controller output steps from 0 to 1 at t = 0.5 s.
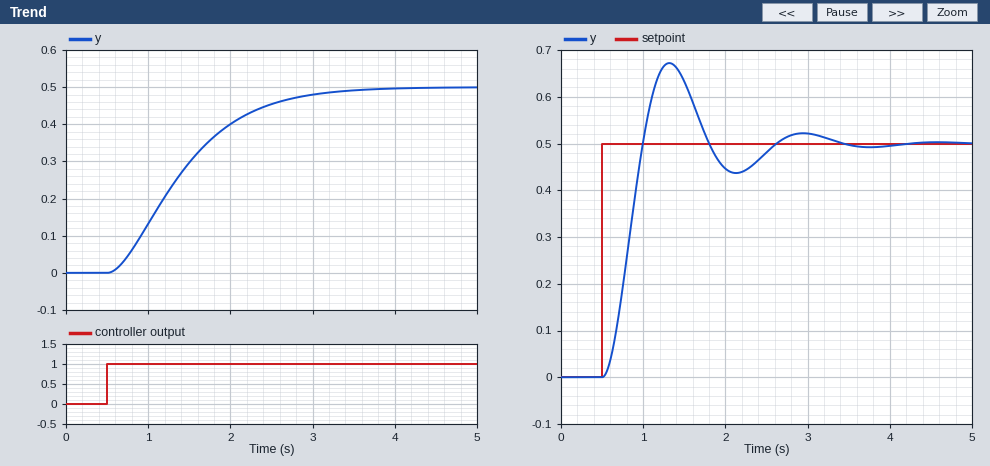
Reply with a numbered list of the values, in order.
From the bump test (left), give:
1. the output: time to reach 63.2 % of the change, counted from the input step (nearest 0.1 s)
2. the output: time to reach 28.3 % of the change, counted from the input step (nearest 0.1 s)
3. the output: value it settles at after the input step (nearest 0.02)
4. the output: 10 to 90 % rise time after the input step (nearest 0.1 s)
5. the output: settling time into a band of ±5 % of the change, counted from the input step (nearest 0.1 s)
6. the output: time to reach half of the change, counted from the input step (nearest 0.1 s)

1. 1.1 s
2. 0.5 s
3. 0.50
4. 1.7 s
5. 2.4 s
6. 0.8 s
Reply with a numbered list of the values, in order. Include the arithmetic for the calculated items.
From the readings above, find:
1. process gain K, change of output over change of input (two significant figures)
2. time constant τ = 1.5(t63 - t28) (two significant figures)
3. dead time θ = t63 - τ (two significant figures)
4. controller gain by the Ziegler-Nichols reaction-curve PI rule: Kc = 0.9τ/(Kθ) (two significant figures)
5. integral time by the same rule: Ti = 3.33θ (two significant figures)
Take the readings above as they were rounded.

1. (0.5 - 0) / 1 = 0.50
2. 1.5 × (1.1 - 0.5) = 0.90 s
3. 1.1 - 0.9 = 0.20 s
4. 0.9 × 0.9 / (0.5 × 0.2) = 8.1
5. 3.33 × 0.2 = 0.67 s
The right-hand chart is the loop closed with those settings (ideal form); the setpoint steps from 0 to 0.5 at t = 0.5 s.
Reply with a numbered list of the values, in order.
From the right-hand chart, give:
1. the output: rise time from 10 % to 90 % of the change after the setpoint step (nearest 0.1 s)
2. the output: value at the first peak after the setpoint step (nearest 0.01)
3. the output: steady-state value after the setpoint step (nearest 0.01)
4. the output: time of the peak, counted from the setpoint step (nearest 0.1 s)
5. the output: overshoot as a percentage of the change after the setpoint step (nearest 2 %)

1. 0.3 s
2. 0.67
3. 0.50
4. 0.8 s
5. 34 %
